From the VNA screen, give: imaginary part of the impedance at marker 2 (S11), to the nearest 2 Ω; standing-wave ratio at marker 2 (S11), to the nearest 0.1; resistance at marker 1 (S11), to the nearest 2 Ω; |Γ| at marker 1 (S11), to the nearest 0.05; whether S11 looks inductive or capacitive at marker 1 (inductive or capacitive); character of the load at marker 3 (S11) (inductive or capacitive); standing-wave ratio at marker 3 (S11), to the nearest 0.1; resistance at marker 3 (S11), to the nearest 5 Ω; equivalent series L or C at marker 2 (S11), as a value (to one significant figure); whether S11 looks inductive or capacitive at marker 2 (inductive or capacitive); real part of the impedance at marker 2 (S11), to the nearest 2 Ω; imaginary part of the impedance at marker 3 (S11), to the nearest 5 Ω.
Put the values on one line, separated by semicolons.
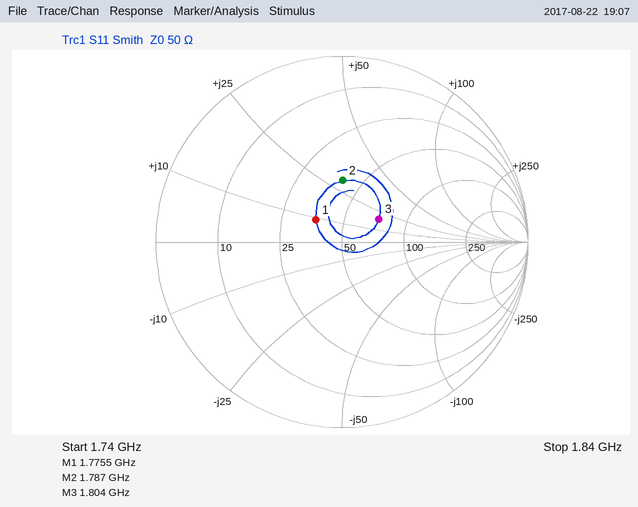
+30 Ω; 2.0; 36 Ω; 0.20; inductive; inductive; 1.6; 70 Ω; 3 nH; inductive; 40 Ω; +20 Ω
